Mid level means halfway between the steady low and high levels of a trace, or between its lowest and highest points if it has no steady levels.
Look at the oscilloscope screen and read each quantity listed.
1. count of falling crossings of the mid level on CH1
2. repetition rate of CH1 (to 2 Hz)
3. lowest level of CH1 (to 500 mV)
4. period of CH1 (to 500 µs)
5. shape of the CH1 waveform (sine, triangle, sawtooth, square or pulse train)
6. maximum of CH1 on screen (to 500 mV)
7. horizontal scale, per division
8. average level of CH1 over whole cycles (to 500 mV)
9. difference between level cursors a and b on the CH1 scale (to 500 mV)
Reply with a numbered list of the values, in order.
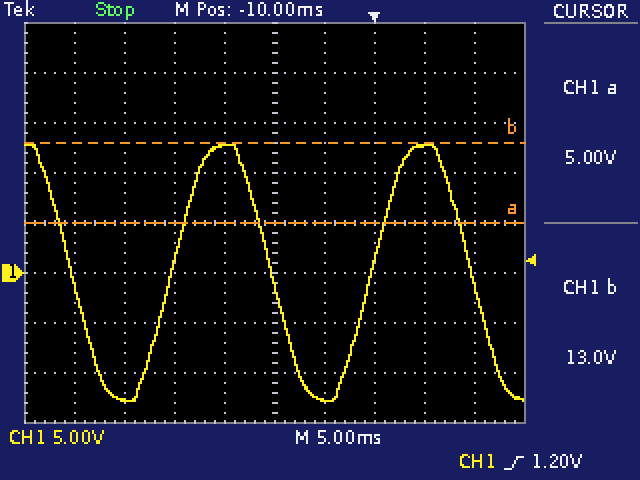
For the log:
1. 3
2. 50 Hz
3. -13.0 V
4. 20.0 ms
5. sine
6. 13.0 V
7. 5 ms
8. 0.0 V
9. 8.0 V
